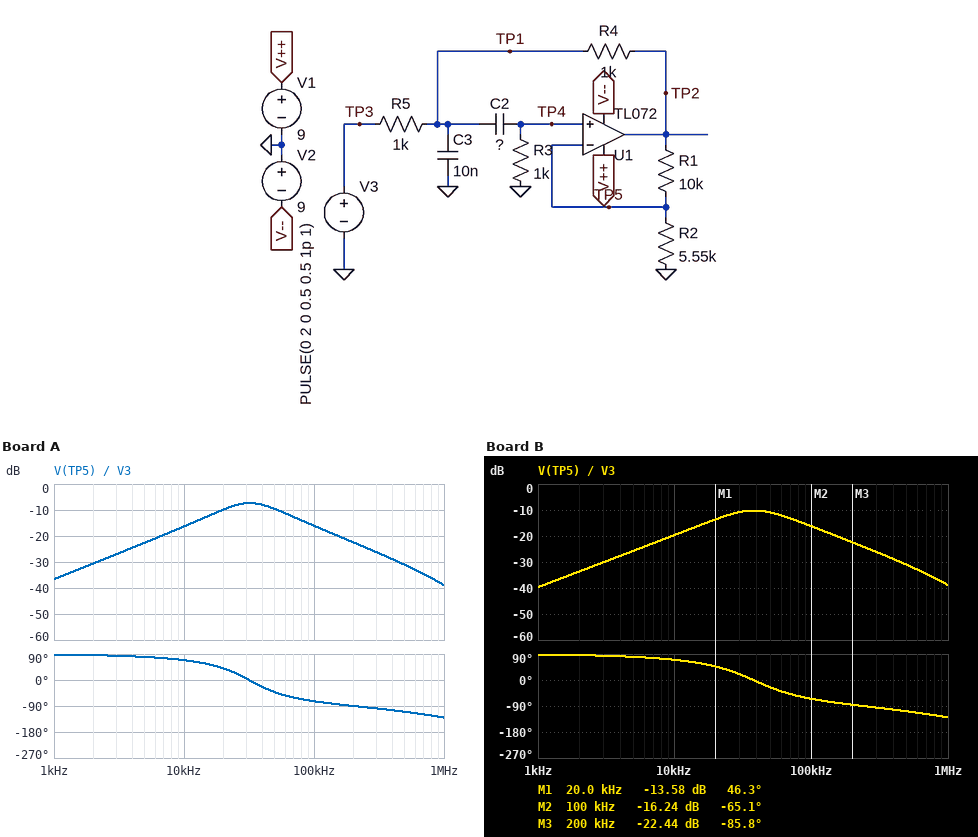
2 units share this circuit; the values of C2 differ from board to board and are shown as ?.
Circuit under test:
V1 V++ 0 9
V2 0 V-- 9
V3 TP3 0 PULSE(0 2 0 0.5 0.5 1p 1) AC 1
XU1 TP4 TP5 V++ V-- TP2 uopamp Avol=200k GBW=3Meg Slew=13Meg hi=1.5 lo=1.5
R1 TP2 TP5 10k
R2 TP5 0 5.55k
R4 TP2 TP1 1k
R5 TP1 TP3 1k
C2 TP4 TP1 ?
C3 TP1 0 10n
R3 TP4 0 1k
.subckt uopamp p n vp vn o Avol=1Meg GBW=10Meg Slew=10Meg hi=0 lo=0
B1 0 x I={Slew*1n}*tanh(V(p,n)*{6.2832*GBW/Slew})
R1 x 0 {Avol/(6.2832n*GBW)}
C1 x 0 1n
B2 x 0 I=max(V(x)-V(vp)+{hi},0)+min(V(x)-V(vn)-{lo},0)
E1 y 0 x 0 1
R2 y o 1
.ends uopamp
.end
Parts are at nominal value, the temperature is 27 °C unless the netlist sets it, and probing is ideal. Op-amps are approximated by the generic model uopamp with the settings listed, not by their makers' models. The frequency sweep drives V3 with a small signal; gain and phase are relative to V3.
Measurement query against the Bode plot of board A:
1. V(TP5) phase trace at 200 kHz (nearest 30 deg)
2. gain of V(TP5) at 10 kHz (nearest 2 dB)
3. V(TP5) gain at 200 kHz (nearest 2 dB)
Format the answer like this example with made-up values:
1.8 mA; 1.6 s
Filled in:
-90 deg; -16 dB; -22 dB
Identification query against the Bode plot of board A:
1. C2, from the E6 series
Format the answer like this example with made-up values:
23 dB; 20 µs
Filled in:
4.7 nF
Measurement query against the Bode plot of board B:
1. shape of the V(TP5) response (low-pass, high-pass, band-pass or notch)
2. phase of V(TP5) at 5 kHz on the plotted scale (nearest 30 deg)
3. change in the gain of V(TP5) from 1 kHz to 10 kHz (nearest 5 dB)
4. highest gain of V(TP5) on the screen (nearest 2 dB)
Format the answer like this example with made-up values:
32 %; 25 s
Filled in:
band-pass; 90 deg; 20 dB; -10 dB
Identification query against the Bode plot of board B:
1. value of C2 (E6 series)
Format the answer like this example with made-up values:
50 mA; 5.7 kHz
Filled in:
3.3 nF
